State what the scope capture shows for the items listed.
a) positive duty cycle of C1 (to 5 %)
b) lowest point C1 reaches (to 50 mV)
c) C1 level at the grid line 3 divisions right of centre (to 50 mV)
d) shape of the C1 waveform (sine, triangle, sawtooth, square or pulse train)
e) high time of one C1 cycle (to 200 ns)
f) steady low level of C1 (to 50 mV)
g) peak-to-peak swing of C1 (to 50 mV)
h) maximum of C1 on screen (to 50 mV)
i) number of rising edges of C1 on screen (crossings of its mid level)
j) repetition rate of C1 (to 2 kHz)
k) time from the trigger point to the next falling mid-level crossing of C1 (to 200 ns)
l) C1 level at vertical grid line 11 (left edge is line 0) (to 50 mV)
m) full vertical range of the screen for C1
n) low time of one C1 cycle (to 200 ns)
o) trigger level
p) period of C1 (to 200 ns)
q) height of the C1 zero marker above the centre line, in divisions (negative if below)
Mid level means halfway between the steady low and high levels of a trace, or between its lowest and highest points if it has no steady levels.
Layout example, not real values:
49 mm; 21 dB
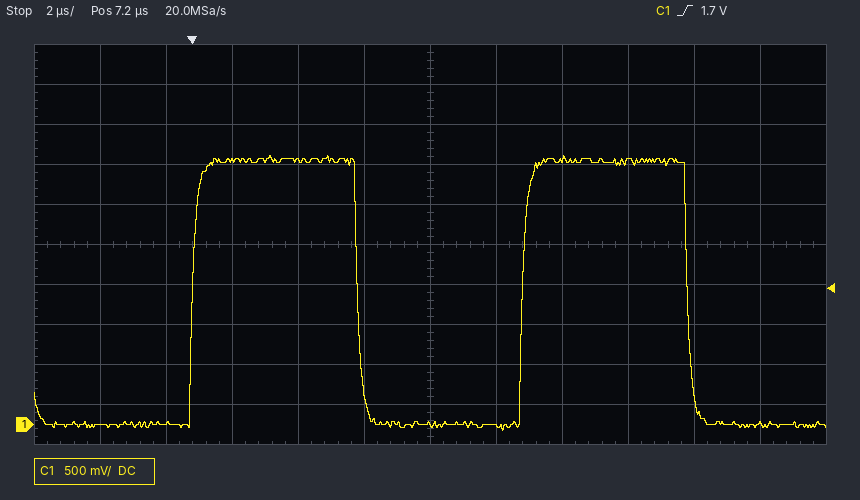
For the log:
50 %; -100 mV; 3.30 V; square; 5.0 µs; 0 mV; 3.45 V; 3.35 V; 2; 100 kHz; 5.0 µs; 0 mV; 5 V; 5.0 µs; 1.7 V; 10.0 µs; -4.5 div
